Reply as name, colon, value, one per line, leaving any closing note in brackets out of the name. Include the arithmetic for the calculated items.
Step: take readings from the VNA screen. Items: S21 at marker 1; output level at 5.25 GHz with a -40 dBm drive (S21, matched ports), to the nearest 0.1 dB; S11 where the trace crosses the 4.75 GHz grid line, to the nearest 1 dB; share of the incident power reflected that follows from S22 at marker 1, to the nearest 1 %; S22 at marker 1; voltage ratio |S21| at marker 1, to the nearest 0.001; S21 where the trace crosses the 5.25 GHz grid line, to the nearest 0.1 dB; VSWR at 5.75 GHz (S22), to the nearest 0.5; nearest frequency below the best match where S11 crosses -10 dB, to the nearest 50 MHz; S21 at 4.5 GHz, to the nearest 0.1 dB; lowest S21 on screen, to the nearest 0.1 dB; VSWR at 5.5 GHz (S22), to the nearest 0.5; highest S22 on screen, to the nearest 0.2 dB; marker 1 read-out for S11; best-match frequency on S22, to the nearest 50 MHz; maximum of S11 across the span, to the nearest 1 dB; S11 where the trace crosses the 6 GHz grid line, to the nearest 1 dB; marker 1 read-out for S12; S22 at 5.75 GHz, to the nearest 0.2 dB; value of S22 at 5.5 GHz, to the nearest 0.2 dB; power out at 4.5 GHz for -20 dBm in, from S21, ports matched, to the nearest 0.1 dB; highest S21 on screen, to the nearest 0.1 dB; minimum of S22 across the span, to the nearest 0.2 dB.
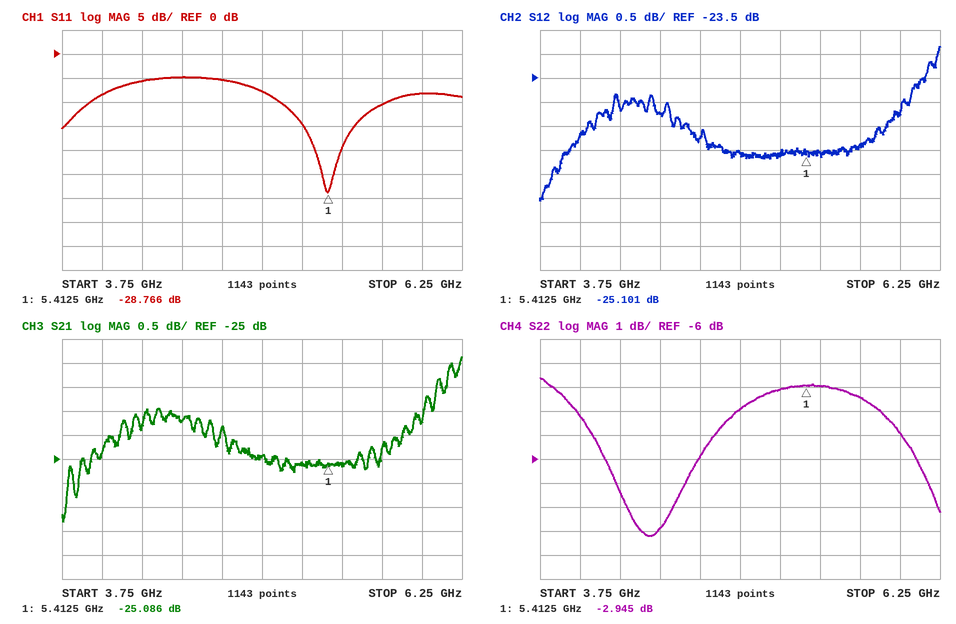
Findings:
S21 at marker 1: -25.086 dB
output level at 5.25 GHz with a -40 dBm drive (S21, matched ports), to the nearest 0.1 dB: -40 dBm + (-25.1 dB) = -65.1 dBm
S11 where the trace crosses the 4.75 GHz grid line, to the nearest 1 dB: -5 dB
share of the incident power reflected that follows from S22 at marker 1, to the nearest 1 %: 10^(-2.945/10) ≈ 51 %
S22 at marker 1: -2.945 dB
voltage ratio |S21| at marker 1, to the nearest 0.001: 10^(-25.086/20) ≈ 0.056
S21 where the trace crosses the 5.25 GHz grid line, to the nearest 0.1 dB: -25.1 dB
VSWR at 5.75 GHz (S22), to the nearest 0.5: |Γ| = 10^(-3.4/20) = 0.6761; VSWR = (1 + 0.6761)/(1 − 0.6761) ≈ 5.17, so 5.0 to the nearest 0.5
nearest frequency below the best match where S11 crosses -10 dB, to the nearest 50 MHz: 5.10 GHz
S21 at 4.5 GHz, to the nearest 0.1 dB: -24.2 dB
lowest S21 on screen, to the nearest 0.1 dB: -26.3 dB
VSWR at 5.5 GHz (S22), to the nearest 0.5: |Γ| = 10^(-3/20) = 0.7079; VSWR = (1 + 0.7079)/(1 − 0.7079) ≈ 5.85, so 6.0 to the nearest 0.5
highest S22 on screen, to the nearest 0.2 dB: -2.6 dB
marker 1 read-out for S11: -28.766 dB
best-match frequency on S22, to the nearest 50 MHz: 4.45 GHz
maximum of S11 across the span, to the nearest 1 dB: -5 dB
S11 where the trace crosses the 6 GHz grid line, to the nearest 1 dB: -8 dB
marker 1 read-out for S12: -25.101 dB
S22 at 5.75 GHz, to the nearest 0.2 dB: -3.4 dB
value of S22 at 5.5 GHz, to the nearest 0.2 dB: -3.0 dB
power out at 4.5 GHz for -20 dBm in, from S21, ports matched, to the nearest 0.1 dB: -20 dBm + (-24.2 dB) = -44.2 dBm
highest S21 on screen, to the nearest 0.1 dB: -22.9 dB
minimum of S22 across the span, to the nearest 0.2 dB: -9.2 dB
